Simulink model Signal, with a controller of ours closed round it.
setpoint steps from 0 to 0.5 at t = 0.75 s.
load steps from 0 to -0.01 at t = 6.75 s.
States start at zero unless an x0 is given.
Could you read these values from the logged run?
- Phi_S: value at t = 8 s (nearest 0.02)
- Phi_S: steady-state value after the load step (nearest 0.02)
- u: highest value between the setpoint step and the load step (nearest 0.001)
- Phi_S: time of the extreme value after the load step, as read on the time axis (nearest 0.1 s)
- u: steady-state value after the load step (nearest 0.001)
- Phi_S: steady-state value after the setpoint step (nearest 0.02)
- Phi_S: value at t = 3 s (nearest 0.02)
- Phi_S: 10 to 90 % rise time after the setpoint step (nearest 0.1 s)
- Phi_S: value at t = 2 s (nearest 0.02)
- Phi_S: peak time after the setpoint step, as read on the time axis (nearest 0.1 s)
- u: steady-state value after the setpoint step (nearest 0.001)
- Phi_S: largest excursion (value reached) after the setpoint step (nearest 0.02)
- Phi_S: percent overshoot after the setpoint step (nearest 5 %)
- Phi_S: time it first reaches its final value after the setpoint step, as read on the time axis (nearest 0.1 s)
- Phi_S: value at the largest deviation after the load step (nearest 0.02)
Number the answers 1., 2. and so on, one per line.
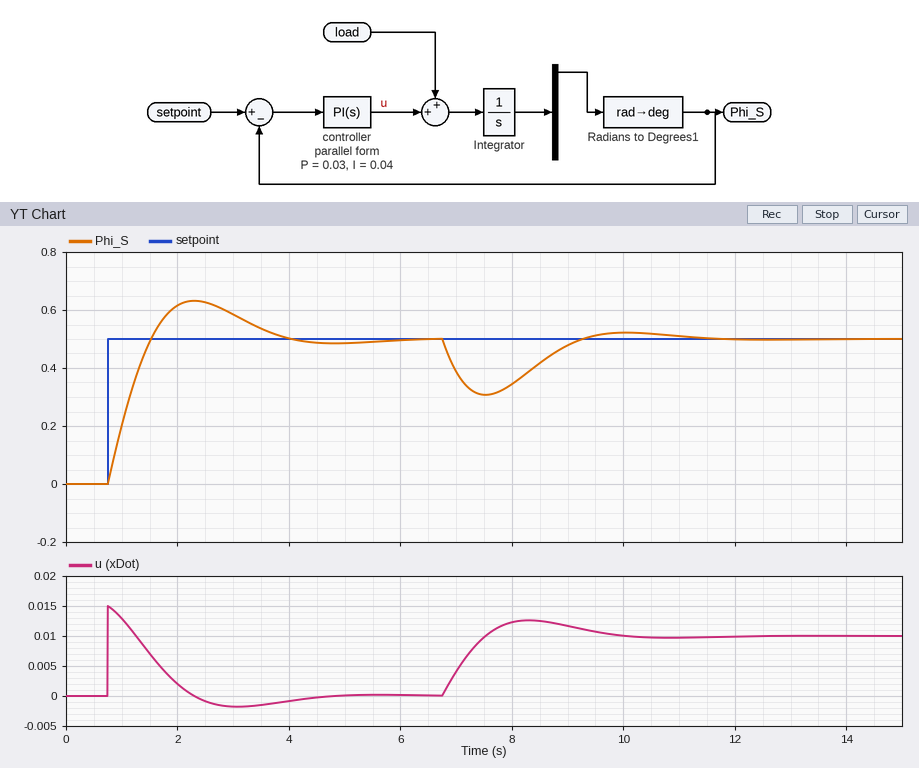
1. 0.34
2. 0.50
3. 0.015
4. 7.5 s
5. 0.010
6. 0.50
7. 0.58
8. 0.6 s
9. 0.62
10. 2.3 s
11. 0.000
12. 0.64
13. 25 %
14. 1.5 s
15. 0.30
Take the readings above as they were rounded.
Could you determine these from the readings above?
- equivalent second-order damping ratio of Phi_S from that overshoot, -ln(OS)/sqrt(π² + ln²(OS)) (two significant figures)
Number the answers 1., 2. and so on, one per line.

1. 0.40
